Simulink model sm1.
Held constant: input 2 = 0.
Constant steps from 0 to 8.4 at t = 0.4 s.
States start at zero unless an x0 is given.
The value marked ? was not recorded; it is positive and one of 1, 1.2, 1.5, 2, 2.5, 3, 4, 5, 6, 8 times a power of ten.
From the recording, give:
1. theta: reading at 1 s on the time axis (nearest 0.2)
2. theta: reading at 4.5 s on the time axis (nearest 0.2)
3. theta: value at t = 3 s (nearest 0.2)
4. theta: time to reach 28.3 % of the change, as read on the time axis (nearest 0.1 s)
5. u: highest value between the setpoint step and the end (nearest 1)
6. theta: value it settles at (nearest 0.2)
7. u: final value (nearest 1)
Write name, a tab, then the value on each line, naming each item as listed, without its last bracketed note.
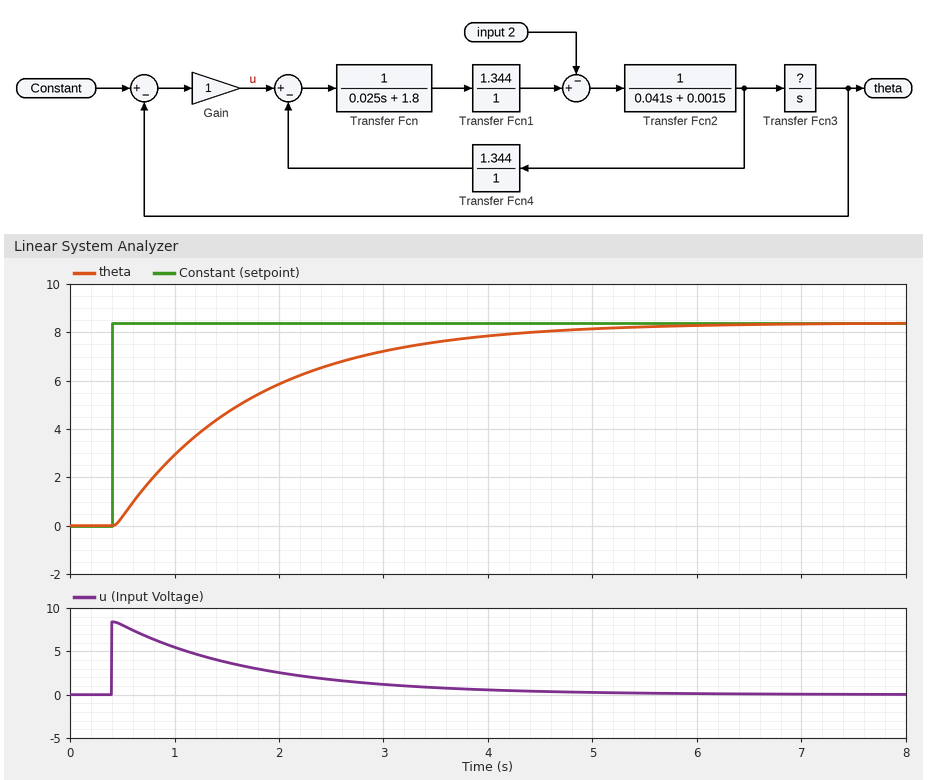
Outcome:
theta: reading at 1 s on the time axis	3.0
theta: reading at 4.5 s on the time axis	8.0
theta: value at t = 3 s	7.2
theta: time to reach 28.3 % of the change, as read on the time axis	0.9 s
u: highest value between the setpoint step and the end	8
theta: value it settles at	8.4
u: final value	0
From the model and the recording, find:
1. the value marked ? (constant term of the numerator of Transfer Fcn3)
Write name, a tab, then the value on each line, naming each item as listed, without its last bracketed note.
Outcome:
the value marked ?	1
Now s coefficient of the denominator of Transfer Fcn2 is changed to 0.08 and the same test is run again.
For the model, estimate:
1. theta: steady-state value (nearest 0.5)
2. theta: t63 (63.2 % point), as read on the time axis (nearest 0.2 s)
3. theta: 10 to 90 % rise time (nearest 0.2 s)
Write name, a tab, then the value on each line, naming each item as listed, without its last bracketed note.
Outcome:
theta: steady-state value	8.5
theta: t63 (63.2 % point), as read on the time axis	1.8 s
theta: 10 to 90 % rise time	2.8 s
